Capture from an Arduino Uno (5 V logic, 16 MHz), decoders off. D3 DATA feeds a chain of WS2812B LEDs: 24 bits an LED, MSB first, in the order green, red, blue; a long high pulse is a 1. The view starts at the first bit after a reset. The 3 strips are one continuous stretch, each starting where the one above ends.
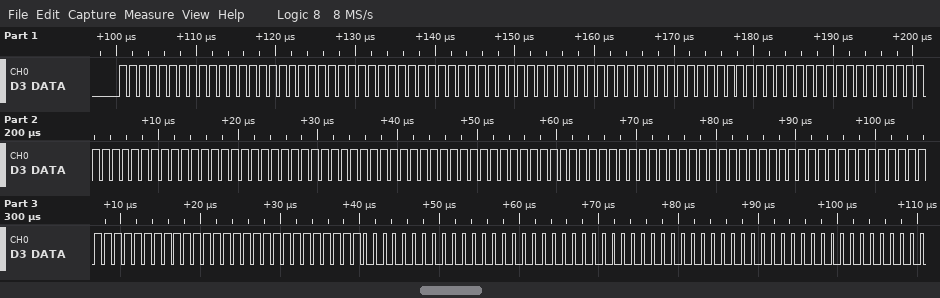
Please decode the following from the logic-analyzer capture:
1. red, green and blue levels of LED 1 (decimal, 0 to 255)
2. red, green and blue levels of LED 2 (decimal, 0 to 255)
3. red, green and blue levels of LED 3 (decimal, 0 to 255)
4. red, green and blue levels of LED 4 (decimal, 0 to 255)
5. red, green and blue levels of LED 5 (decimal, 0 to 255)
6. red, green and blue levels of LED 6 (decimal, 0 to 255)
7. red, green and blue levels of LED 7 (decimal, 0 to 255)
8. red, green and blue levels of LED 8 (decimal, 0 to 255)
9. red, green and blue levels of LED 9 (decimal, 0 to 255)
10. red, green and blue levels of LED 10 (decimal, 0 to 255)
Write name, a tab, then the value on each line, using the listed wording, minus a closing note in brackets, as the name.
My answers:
red, green and blue levels of LED 1	255, 255, 255
red, green and blue levels of LED 2	255, 255, 255
red, green and blue levels of LED 3	255, 255, 255
red, green and blue levels of LED 4	255, 255, 255
red, green and blue levels of LED 5	255, 255, 255
red, green and blue levels of LED 6	255, 255, 255
red, green and blue levels of LED 7	255, 255, 255
red, green and blue levels of LED 8	255, 255, 255
red, green and blue levels of LED 9	0, 0, 0
red, green and blue levels of LED 10	0, 0, 0
